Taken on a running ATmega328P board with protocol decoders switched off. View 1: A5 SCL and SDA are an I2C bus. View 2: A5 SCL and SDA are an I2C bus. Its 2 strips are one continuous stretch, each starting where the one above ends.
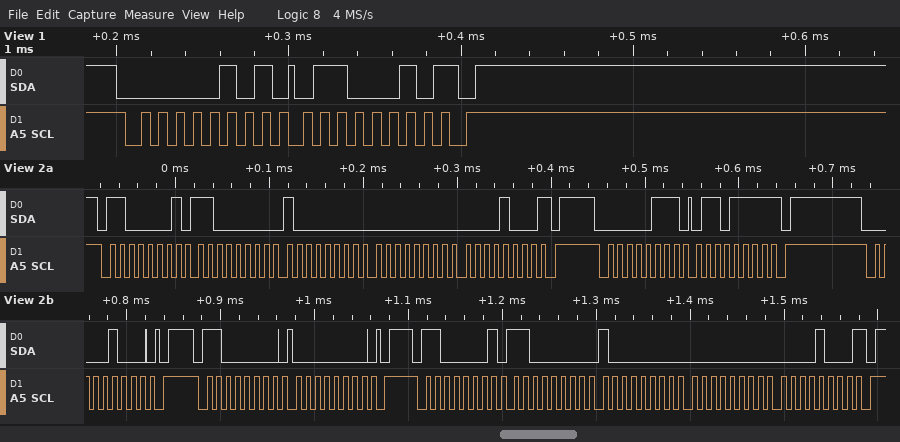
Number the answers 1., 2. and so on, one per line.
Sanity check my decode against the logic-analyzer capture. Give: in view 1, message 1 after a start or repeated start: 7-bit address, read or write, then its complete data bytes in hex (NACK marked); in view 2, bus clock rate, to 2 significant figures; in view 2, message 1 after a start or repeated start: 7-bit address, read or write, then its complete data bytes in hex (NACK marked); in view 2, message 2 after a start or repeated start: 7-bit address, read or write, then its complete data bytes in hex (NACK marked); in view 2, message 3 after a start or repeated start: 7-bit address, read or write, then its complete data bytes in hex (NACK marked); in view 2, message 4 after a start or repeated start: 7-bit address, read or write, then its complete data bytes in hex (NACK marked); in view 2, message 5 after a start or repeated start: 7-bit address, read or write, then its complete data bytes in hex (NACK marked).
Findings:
1. 0x02 read: 62 NACK
2. 100 kHz
3. 0x60 read: C0 80 00 08 NACK
4. 0x03 read: 6F NACK
5. 0x04 write
6. 0x60 write: 00
7. 0x60 read: C0 80 00 08 NACK
